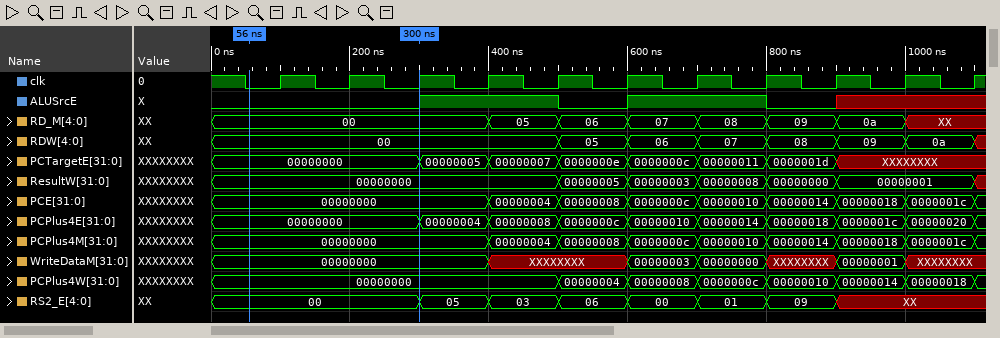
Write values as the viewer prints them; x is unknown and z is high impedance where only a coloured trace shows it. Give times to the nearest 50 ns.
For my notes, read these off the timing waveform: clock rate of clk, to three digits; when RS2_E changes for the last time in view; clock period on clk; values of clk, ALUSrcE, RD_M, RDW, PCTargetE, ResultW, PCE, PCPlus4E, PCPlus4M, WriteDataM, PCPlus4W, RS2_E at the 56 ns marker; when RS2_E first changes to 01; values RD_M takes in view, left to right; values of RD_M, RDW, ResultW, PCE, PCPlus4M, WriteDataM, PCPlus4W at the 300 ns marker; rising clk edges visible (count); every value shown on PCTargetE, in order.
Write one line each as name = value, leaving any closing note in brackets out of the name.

clock rate of clk, to three digits = 10.0 MHz
when RS2_E changes for the last time in view = 900 ns
clock period on clk = 100 ns
values of clk, ALUSrcE, RD_M, RDW, PCTargetE, ResultW, PCE, PCPlus4E, PCPlus4M, WriteDataM, PCPlus4W, RS2_E at the 56 ns marker = clk=0, ALUSrcE=0, RD_M=00, RDW=00, PCTargetE=00000000, ResultW=00000000, PCE=00000000, PCPlus4E=00000000, PCPlus4M=00000000, WriteDataM=00000000, PCPlus4W=00000000, RS2_E=00
when RS2_E first changes to 01 = 700 ns
values RD_M takes in view, left to right = 00, 05, 06, 07, 08, 09, 0a, XX
values of RD_M, RDW, ResultW, PCE, PCPlus4M, WriteDataM, PCPlus4W at the 300 ns marker = RD_M=00, RDW=00, ResultW=00000000, PCE=00000000, PCPlus4M=00000000, WriteDataM=00000000, PCPlus4W=00000000
rising clk edges visible = 11
every value shown on PCTargetE, in order = 00000000, 00000005, 00000007, 0000000e, 0000000c, 00000011, 0000001d, XXXXXXXX
